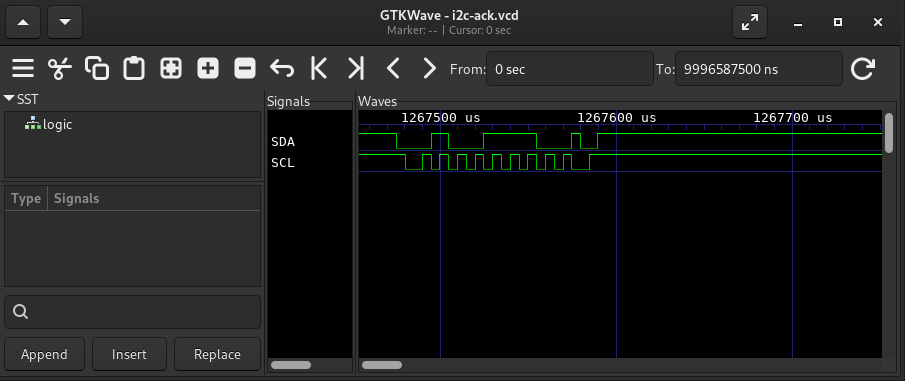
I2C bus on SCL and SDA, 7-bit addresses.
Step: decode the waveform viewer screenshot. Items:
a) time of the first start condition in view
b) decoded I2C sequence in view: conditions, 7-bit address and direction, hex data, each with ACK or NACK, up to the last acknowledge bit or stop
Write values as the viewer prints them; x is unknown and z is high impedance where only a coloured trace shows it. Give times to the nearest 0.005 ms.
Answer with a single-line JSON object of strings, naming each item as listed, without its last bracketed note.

{"time of the first start condition in view": "1267.475 ms", "decoded I2C sequence in view: conditions, 7-bit address and direction, hex data, each with ACK or NACK, up to the last acknowledge bit or stop": "start, address 27 write ACK, stop"}
